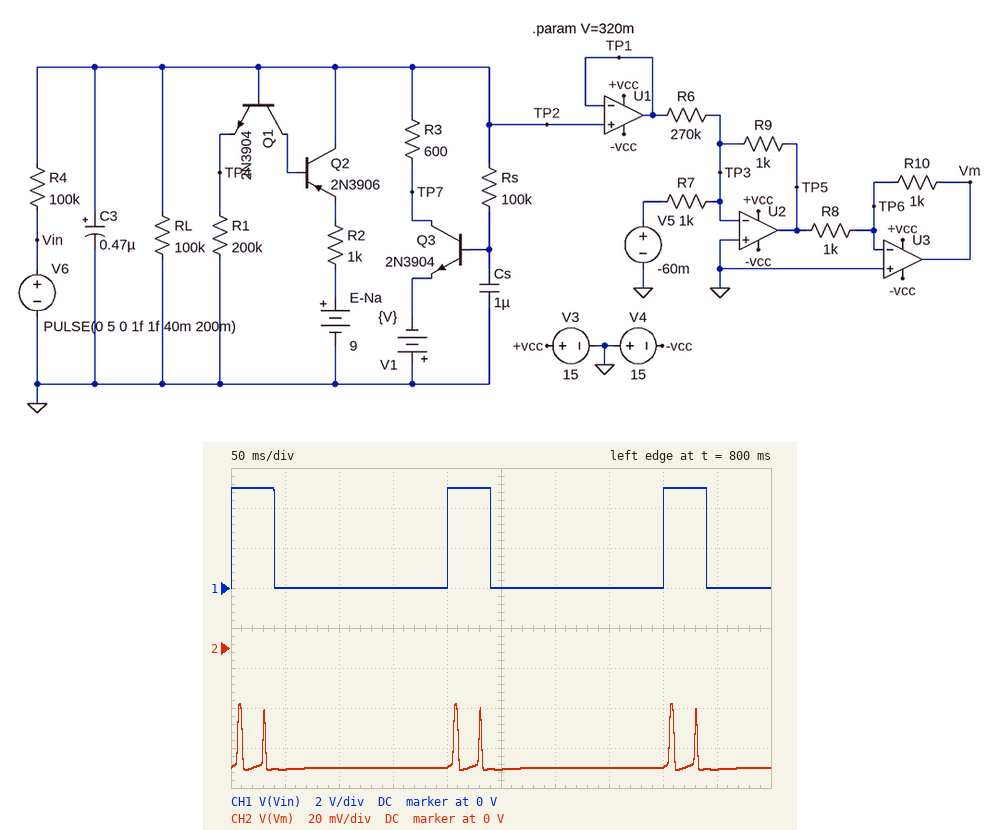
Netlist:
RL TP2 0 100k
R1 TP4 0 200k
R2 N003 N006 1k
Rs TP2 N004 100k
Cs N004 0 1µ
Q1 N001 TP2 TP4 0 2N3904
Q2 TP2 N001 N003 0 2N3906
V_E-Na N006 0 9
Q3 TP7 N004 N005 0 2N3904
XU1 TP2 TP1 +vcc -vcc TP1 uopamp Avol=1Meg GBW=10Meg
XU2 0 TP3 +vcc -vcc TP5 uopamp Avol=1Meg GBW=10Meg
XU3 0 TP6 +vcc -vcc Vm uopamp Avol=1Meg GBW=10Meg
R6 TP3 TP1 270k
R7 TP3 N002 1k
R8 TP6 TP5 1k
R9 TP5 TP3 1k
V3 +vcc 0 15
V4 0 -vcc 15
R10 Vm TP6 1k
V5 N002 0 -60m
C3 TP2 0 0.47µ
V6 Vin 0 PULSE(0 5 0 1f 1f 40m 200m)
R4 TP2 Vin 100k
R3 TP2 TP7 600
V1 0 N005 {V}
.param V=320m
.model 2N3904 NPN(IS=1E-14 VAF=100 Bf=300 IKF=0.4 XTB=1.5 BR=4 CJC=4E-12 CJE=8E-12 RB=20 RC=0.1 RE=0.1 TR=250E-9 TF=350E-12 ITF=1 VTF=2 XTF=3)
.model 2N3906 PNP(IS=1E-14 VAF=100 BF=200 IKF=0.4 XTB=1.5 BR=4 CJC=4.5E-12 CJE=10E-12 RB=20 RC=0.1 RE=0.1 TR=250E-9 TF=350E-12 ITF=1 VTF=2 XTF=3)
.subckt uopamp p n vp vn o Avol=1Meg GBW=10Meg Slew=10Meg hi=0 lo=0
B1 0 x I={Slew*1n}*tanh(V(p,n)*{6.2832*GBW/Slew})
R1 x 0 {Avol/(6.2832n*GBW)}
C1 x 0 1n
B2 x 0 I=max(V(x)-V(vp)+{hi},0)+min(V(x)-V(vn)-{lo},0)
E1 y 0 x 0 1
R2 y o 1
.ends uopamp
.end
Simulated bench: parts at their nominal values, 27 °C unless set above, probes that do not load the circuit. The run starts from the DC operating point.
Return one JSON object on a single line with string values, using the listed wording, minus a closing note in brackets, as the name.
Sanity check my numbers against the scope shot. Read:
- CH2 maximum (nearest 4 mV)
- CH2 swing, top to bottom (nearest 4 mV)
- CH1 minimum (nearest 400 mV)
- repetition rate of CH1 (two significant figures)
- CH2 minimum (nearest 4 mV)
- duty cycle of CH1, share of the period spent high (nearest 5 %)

{"CH2 maximum": "-28 mV", "CH2 swing, top to bottom": "32 mV", "CH1 minimum": "0 V", "repetition rate of CH1": "5.0 Hz", "CH2 minimum": "-60 mV", "duty cycle of CH1, share of the period spent high": "20 %"}
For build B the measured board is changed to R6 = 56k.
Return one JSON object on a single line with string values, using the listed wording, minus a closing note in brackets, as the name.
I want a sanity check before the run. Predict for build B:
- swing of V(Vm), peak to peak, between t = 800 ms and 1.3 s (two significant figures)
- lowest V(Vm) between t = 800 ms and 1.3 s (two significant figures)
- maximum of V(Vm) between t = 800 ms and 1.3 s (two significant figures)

{"swing of V(Vm), peak to peak, between t = 800 ms and 1.3 s": "160 mV", "lowest V(Vm) between t = 800 ms and 1.3 s": "-65 mV", "maximum of V(Vm) between t = 800 ms and 1.3 s": "95 mV"}
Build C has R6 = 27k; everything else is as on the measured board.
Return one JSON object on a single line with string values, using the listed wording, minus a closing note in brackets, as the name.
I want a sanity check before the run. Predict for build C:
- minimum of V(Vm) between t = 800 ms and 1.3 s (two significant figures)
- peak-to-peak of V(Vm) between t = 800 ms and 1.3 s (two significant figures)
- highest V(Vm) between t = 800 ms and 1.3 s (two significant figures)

{"minimum of V(Vm) between t = 800 ms and 1.3 s": "-70 mV", "peak-to-peak of V(Vm) between t = 800 ms and 1.3 s": "330 mV", "highest V(Vm) between t = 800 ms and 1.3 s": "260 mV"}
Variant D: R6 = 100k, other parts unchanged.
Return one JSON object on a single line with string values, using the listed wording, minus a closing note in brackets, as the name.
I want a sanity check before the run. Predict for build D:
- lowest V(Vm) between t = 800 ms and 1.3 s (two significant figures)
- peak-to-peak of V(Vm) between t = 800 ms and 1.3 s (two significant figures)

{"lowest V(Vm) between t = 800 ms and 1.3 s": "-63 mV", "peak-to-peak of V(Vm) between t = 800 ms and 1.3 s": "89 mV"}
